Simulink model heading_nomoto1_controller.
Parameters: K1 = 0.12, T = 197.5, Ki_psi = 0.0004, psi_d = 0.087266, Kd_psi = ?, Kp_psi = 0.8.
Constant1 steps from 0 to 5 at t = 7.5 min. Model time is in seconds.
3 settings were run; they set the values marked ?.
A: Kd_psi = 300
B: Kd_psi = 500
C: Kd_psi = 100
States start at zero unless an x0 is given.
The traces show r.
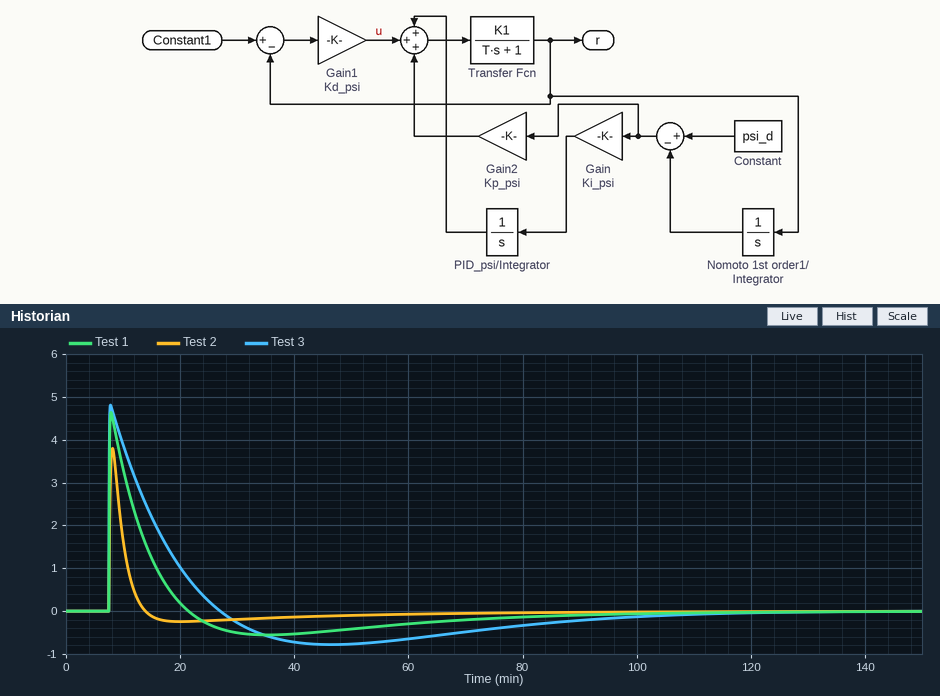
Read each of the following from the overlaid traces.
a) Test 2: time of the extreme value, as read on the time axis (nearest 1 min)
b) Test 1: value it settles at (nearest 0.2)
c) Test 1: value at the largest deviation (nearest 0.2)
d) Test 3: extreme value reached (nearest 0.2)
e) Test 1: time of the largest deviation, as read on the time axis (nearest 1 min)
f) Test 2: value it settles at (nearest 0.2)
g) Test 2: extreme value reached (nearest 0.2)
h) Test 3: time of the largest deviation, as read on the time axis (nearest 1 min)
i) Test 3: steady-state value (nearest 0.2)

8 min
0.0
4.6
4.8
8 min
0.0
3.8
8 min
0.0
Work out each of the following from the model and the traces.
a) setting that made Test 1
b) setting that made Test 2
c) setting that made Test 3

A
C
B
